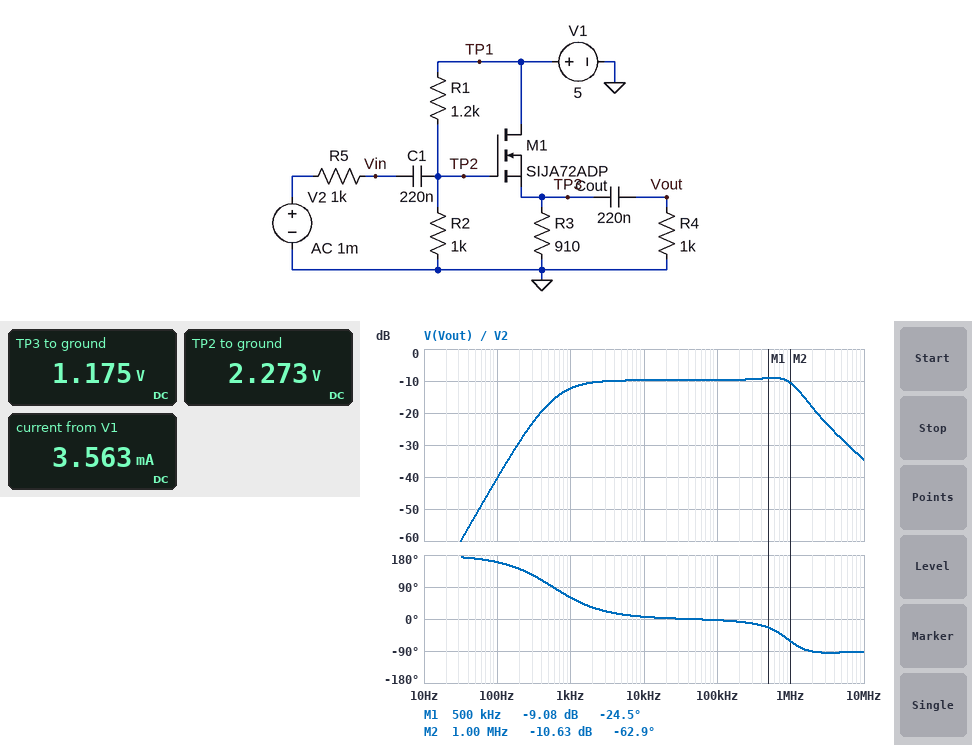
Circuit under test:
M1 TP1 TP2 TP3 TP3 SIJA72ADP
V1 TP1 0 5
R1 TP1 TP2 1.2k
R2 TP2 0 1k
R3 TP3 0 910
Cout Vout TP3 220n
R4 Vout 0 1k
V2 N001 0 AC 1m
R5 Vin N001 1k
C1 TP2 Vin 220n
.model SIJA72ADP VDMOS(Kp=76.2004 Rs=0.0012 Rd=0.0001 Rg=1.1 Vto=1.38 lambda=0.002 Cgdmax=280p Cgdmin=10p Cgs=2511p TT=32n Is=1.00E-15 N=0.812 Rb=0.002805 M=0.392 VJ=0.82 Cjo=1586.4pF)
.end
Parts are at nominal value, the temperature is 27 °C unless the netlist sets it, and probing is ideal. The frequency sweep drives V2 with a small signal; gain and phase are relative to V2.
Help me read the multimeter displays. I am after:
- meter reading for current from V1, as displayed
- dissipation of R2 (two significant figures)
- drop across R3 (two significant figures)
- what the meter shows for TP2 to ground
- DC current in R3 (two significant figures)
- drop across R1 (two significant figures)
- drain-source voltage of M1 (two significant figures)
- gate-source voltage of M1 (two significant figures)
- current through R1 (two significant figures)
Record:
3.563 mA
5.2 mW
1.2 V
2.273 V
1.3 mA
2.7 V
3.8 V
1.1 V
2.3 mA
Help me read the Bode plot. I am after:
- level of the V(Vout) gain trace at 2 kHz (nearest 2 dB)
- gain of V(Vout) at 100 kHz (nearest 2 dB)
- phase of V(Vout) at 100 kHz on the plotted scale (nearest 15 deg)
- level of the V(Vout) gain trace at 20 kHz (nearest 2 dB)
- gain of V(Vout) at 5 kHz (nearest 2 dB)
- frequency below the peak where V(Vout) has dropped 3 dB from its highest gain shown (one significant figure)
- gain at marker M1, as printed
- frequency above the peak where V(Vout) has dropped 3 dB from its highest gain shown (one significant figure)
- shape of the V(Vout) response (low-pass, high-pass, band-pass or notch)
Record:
-10 dB
-10 dB
0 deg
-10 dB
-10 dB
1 kHz
-9.08 dB
1 MHz
band-pass
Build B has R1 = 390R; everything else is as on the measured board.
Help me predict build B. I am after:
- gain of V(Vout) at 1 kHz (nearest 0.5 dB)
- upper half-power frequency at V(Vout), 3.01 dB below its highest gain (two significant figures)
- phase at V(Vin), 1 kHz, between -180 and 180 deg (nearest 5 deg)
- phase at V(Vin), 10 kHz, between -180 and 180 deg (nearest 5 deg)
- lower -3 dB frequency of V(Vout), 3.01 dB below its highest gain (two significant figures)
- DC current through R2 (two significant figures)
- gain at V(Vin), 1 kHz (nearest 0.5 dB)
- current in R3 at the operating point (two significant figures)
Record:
-16.5 dB
1.9 MHz
-40 deg
-10 deg
1.6 kHz
3.6 mA
-5.5 dB
2.7 mA
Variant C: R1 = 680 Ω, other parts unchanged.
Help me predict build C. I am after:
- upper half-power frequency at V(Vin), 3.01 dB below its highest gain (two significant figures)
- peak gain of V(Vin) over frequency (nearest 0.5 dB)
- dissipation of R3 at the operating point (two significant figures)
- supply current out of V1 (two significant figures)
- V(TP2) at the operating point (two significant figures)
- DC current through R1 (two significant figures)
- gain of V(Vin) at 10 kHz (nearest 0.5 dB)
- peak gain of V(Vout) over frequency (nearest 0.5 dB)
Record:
560 Hz
0 dB
3.8 mW
5.0 mA
3.0 V
3.0 mA
-10.5 dB
-10.0 dB
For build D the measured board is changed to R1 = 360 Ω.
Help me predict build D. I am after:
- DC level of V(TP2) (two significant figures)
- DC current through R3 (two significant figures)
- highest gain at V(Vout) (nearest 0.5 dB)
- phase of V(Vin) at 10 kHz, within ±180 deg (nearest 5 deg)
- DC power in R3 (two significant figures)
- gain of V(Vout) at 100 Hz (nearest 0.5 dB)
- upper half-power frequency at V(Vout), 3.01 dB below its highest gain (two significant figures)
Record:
3.7 V
2.8 mA
-12.0 dB
-10 deg
7.1 mW
-46.5 dB
2.0 MHz
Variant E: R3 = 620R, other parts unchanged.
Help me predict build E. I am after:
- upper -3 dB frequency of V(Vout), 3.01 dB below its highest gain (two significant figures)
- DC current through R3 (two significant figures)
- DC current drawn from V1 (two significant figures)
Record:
1.4 MHz
1.9 mA
4.1 mA
